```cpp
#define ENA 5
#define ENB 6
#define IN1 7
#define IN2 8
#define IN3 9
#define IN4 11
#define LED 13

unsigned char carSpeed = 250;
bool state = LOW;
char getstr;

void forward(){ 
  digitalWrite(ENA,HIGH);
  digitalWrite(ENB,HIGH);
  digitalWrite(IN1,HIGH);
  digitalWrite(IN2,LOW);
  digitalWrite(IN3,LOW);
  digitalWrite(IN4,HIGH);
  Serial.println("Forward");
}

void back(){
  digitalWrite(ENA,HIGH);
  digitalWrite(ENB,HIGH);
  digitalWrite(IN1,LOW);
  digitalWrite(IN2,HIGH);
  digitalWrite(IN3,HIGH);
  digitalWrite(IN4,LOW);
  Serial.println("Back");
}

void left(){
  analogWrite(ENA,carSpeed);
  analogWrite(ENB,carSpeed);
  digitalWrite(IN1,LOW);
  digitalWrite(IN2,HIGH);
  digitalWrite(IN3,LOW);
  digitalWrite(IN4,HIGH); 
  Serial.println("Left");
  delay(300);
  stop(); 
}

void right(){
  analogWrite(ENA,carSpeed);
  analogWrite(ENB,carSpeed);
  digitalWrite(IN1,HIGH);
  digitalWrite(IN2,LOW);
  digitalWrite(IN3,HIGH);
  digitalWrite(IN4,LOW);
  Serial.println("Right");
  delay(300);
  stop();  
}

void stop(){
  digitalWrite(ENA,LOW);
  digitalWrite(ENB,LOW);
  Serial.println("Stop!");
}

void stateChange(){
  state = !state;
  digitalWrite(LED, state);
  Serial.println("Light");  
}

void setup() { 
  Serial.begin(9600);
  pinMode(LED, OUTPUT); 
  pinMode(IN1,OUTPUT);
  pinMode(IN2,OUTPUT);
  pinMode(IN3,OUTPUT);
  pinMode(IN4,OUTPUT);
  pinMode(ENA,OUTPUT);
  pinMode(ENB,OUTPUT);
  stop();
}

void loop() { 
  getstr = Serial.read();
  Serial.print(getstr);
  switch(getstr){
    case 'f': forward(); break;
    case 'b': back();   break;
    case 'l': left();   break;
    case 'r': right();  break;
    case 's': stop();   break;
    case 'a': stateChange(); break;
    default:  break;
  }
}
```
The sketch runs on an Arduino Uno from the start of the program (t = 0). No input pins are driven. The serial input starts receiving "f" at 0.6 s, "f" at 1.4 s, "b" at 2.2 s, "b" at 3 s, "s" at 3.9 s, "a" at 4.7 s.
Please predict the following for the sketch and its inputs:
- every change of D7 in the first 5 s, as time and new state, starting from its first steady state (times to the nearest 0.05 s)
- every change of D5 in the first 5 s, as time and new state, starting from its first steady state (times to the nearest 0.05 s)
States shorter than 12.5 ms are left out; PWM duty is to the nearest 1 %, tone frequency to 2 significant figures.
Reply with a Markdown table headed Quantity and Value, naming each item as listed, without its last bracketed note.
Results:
| Quantity | Value |
|---|---|
| every change of D7 in the first 5 s, as time and new state, starting from its first steady state | 0 s low; 0.6 s high; 2.2 s low |
| every change of D5 in the first 5 s, as time and new state, starting from its first steady state | 0 s low; 0.6 s high; 3.9 s low |
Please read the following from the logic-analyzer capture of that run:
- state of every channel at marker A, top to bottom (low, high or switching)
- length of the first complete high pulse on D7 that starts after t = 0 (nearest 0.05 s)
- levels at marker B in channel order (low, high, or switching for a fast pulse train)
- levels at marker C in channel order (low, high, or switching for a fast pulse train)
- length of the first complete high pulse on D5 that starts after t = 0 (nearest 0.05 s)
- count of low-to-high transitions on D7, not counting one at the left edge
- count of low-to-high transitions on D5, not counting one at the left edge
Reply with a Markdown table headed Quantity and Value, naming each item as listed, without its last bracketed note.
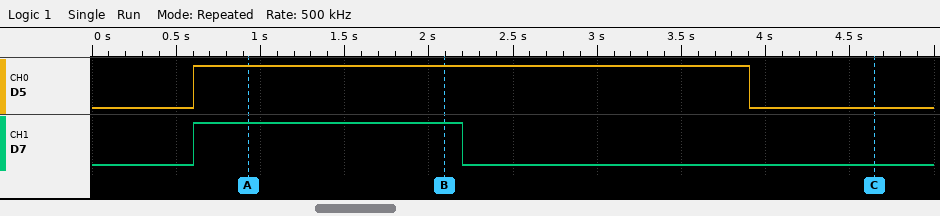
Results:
| Quantity | Value |
|---|---|
| state of every channel at marker A, top to bottom | D5 high, D7 high |
| length of the first complete high pulse on D7 that starts after t = 0 | 1.60 s |
| levels at marker B in channel order | D5 high, D7 high |
| levels at marker C in channel order | D5 low, D7 low |
| length of the first complete high pulse on D5 that starts after t = 0 | 3.30 s |
| count of low-to-high transitions on D7, not counting one at the left edge | 1 |
| count of low-to-high transitions on D5, not counting one at the left edge | 1 |
